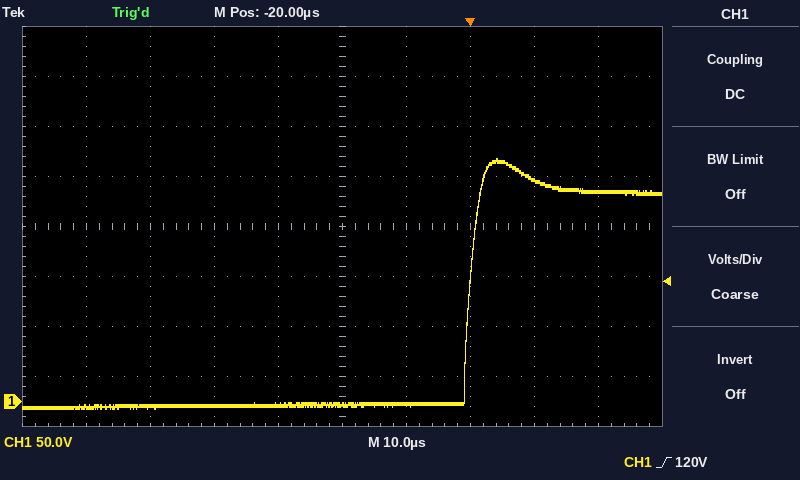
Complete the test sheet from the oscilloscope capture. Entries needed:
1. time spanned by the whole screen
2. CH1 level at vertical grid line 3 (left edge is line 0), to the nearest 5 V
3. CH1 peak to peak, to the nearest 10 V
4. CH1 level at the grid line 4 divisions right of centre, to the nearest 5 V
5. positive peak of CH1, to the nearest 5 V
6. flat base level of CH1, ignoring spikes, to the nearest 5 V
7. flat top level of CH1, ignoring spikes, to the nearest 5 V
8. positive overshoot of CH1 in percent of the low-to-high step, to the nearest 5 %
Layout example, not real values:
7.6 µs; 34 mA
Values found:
100 µs; -5 V; 250 V; 210 V; 245 V; -5 V; 210 V; 15 %
